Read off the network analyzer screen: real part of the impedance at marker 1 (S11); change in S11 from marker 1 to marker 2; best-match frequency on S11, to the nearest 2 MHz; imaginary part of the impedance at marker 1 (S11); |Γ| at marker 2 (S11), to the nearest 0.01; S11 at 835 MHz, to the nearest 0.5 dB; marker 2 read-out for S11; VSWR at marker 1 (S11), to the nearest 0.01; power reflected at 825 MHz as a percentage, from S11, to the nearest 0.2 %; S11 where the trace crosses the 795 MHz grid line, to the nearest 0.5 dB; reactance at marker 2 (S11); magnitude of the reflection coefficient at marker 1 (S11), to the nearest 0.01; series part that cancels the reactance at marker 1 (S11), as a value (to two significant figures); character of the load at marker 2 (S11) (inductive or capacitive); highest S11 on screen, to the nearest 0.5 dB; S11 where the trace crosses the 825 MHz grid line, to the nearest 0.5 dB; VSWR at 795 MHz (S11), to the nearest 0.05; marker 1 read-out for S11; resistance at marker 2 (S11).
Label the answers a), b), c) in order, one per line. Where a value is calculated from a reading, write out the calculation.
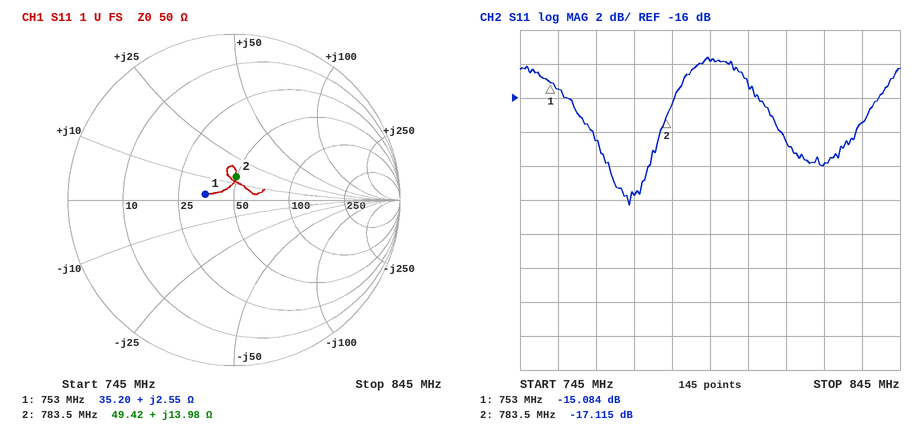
a) 35.20 Ω
b) -17.115 − (-15.084) = -2.031 dB
c) 774 MHz
d) +2.55 Ω
e) 0.14
f) -17.5 dB
g) -17.115 dB
h) (1 + 0.1761)/(1 − 0.1761) ≈ 1.43
i) 10^(-20/10) ≈ 1.0 %
j) -14.0 dB
k) +13.98 Ω
l) 0.18
m) C = 1/(2π × 753 MHz × 2.55 Ω) ≈ 83 pF
n) inductive
o) -13.5 dB
p) -20.0 dB
q) |Γ| = 10^(-14/20) = 0.1995; VSWR = (1 + 0.1995)/(1 − 0.1995) ≈ 1.50
r) -15.084 dB
s) 49.42 Ω
